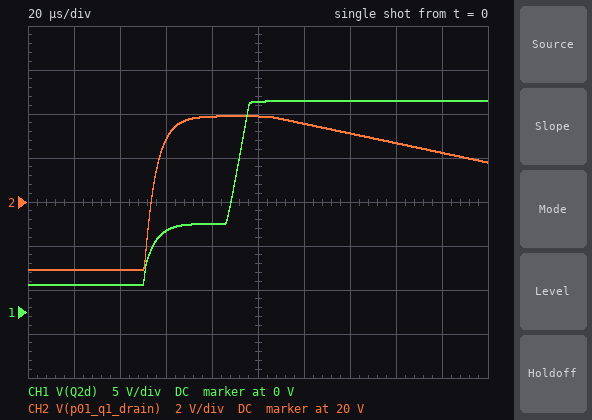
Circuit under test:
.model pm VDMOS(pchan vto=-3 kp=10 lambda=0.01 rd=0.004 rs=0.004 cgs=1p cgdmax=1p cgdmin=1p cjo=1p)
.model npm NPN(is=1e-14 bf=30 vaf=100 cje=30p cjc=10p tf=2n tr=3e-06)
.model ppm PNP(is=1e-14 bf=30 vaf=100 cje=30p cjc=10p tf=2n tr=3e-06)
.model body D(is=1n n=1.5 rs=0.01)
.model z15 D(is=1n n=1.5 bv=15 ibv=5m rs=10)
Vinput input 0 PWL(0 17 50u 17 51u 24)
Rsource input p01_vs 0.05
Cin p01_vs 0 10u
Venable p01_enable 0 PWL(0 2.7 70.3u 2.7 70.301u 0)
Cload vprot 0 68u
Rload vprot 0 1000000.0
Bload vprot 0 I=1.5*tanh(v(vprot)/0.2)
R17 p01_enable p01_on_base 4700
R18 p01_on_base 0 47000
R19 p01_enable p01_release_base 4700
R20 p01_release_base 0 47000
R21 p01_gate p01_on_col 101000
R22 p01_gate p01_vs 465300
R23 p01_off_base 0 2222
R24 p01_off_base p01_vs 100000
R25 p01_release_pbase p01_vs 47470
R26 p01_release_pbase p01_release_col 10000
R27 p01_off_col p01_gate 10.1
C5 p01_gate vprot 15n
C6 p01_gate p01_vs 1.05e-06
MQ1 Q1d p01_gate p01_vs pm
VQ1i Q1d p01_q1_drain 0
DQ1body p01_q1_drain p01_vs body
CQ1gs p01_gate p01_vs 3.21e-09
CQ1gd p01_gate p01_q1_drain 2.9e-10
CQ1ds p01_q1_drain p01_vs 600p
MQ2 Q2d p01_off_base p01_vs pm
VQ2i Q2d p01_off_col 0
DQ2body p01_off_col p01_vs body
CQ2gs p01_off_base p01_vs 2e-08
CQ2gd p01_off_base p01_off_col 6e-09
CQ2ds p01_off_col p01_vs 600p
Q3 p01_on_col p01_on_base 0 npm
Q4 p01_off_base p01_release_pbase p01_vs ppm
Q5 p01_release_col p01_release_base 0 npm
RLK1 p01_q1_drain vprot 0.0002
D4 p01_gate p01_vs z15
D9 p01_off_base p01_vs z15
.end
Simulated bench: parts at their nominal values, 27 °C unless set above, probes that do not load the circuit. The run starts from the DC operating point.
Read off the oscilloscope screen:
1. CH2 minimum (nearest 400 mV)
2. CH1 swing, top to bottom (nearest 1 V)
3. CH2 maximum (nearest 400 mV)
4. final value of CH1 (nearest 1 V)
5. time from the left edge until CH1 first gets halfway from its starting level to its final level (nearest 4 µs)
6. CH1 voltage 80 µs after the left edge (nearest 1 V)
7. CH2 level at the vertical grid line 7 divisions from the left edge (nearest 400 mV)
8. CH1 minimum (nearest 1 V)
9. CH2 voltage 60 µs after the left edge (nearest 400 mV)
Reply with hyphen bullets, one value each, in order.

- 16.8 V
- 21 V
- 24.0 V
- 24 V
- 88 µs
- 10 V
- 23.2 V
- 3 V
- 22.8 V
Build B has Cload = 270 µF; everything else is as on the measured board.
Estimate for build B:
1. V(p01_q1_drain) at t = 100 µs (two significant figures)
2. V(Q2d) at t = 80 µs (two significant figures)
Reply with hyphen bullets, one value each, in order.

- 23 V
- 8.9 V
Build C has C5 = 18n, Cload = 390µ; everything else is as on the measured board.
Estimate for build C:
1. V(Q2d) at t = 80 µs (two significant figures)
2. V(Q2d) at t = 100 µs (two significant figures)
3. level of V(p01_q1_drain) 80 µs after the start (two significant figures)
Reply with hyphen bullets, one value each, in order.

- 8.3 V
- 23 V
- 22 V
